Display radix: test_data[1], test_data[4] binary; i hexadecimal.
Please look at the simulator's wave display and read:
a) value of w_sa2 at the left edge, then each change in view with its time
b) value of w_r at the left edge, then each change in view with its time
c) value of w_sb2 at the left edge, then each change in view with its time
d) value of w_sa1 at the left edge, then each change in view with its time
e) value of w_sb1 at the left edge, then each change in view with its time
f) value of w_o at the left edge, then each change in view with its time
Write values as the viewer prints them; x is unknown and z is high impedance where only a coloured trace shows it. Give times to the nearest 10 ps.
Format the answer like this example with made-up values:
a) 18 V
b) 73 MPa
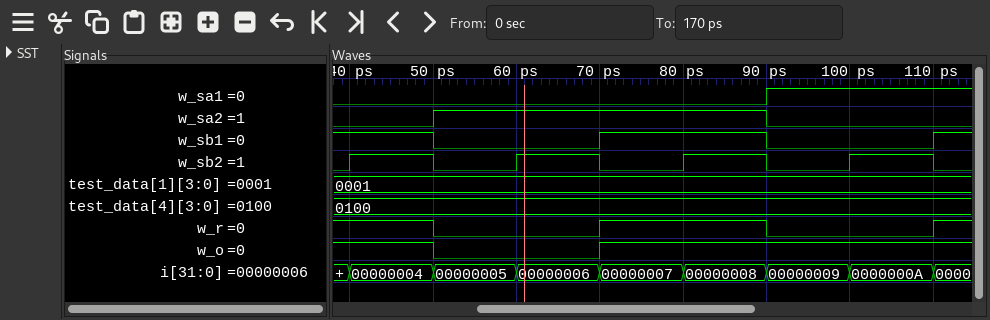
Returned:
a) 0, 1 at 50 ps, 0 at 90 ps
b) 1, 0 at 50 ps, 1 at 70 ps, 0 at 90 ps, 1 at 110 ps
c) 0, 1 at 40 ps, 0 at 50 ps, 1 at 60 ps, 0 at 70 ps, 1 at 80 ps, 0 at 90 ps, 1 at 100 ps, 0 at 110 ps
d) 0, 1 at 90 ps
e) 1, 0 at 50 ps, 1 at 70 ps, 0 at 90 ps, 1 at 110 ps
f) 1, 0 at 50 ps, 1 at 70 ps
